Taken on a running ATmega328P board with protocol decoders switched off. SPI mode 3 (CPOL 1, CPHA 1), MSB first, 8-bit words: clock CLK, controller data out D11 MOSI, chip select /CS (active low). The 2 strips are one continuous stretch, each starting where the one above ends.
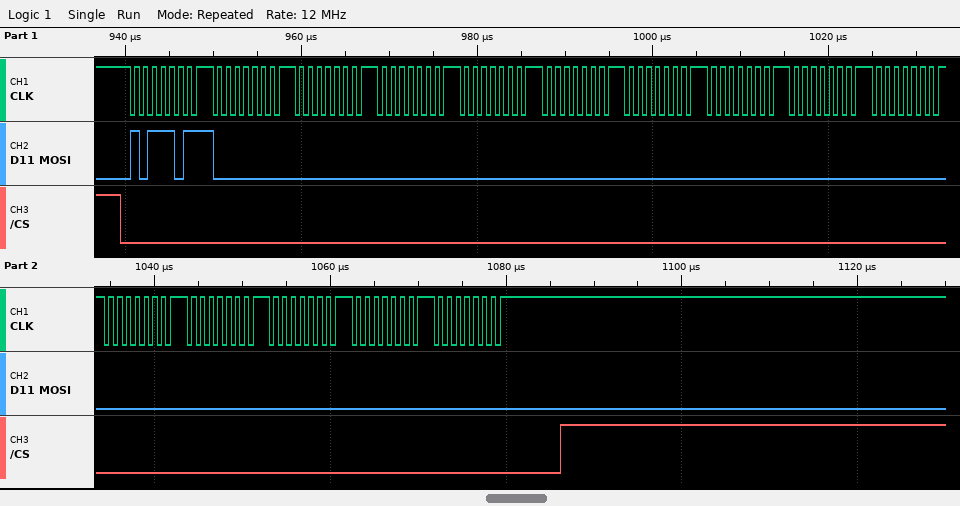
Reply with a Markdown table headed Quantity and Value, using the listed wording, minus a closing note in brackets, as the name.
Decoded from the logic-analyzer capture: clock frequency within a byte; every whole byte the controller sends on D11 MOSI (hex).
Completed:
| Quantity | Value |
|---|---|
| clock frequency within a byte | 1 MHz |
| every whole byte the controller sends on D11 MOSI | 0xBB 0x00 0x00 0x00 0x00 0x00 0x00 0x00 0x00 0x00 0x00 0x00 0x00 0x00 0x00 |
